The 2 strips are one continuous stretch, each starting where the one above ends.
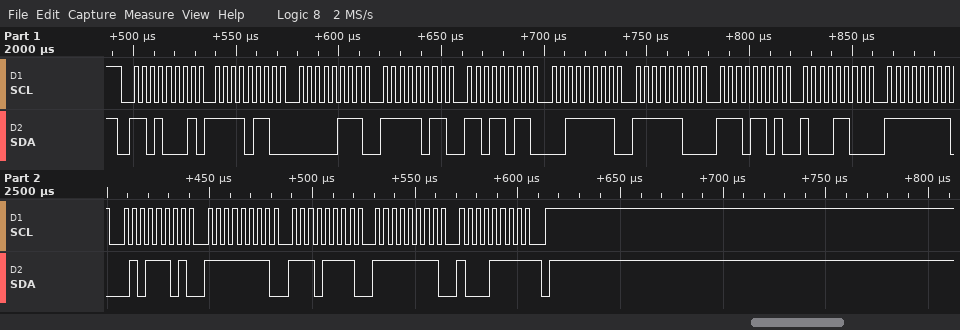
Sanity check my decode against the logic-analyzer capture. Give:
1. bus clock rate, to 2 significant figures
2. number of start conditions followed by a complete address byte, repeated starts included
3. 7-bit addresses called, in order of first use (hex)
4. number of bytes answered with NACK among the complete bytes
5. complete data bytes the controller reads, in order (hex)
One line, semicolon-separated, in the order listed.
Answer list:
250 kHz; 1; 0x68; 1; F6 07 FB DB 3F FC ED 8C FF 5D FF EF FF 8F
